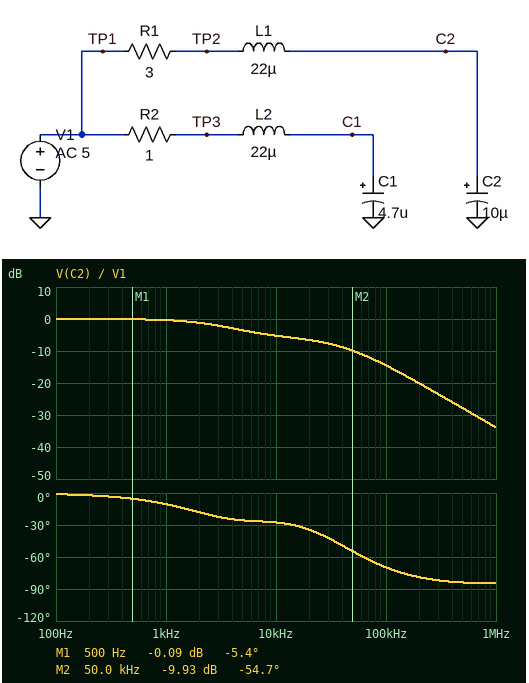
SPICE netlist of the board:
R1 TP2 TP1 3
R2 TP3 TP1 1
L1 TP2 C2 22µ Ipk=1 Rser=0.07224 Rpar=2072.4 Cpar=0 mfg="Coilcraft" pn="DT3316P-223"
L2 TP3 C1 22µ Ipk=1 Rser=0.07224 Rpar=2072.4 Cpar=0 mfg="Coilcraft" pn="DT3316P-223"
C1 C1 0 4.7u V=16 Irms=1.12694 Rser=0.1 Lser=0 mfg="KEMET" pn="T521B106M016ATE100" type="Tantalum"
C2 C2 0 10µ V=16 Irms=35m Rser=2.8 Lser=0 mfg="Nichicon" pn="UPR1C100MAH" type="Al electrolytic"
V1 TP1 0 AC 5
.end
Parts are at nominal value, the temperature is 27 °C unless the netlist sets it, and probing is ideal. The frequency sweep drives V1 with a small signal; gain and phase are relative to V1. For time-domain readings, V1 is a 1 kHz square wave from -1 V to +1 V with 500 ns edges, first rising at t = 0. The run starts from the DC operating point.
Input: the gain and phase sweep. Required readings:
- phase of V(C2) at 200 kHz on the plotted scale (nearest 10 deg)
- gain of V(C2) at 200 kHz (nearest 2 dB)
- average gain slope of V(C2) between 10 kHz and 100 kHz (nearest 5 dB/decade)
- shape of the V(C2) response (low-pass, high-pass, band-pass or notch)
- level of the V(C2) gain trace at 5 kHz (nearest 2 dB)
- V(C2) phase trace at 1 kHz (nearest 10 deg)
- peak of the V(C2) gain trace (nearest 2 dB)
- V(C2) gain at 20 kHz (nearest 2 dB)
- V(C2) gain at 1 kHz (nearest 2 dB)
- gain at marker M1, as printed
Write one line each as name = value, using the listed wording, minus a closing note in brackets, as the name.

phase of V(C2) at 200 kHz on the plotted scale = -80 deg
gain of V(C2) at 200 kHz = -20 dB
average gain slope of V(C2) between 10 kHz and 100 kHz = -10 dB/decade
shape of the V(C2) response = low-pass
level of the V(C2) gain trace at 5 kHz = -4 dB
V(C2) phase trace at 1 kHz = -10 deg
peak of the V(C2) gain trace = 0 dB
V(C2) gain at 20 kHz = -6 dB
V(C2) gain at 1 kHz = 0 dB
gain at marker M1, as printed = -0.09 dB
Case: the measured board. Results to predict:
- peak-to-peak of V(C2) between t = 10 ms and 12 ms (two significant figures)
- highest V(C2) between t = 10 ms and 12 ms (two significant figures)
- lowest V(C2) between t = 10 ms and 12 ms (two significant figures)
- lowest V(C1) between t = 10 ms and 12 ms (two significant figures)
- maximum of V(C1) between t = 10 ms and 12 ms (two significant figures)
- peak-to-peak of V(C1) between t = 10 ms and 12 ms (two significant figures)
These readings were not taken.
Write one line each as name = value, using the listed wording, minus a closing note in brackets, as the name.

peak-to-peak of V(C2) between t = 10 ms and 12 ms = 2.0 V
highest V(C2) between t = 10 ms and 12 ms = 1.0 V
lowest V(C2) between t = 10 ms and 12 ms = -1.0 V
lowest V(C1) between t = 10 ms and 12 ms = -1.8 V
maximum of V(C1) between t = 10 ms and 12 ms = 1.8 V
peak-to-peak of V(C1) between t = 10 ms and 12 ms = 3.7 V
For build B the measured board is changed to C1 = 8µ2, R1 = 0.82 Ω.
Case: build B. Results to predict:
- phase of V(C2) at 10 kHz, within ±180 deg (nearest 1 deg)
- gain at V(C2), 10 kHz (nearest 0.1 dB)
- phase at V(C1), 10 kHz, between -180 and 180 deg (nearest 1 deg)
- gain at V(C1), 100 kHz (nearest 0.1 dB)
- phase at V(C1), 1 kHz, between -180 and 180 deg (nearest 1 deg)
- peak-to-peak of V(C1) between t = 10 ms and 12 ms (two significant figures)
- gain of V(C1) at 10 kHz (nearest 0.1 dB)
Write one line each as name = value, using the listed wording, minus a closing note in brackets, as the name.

phase of V(C2) at 10 kHz, within ±180 deg = -26 deg
gain at V(C2), 10 kHz = -1.2 dB
phase at V(C1), 10 kHz, between -180 and 180 deg = -62 deg
gain at V(C1), 100 kHz = -35.9 dB
phase at V(C1), 1 kHz, between -180 and 180 deg = -3 deg
peak-to-peak of V(C1) between t = 10 ms and 12 ms = 3.2 V
gain of V(C1) at 10 kHz = 3.5 dB
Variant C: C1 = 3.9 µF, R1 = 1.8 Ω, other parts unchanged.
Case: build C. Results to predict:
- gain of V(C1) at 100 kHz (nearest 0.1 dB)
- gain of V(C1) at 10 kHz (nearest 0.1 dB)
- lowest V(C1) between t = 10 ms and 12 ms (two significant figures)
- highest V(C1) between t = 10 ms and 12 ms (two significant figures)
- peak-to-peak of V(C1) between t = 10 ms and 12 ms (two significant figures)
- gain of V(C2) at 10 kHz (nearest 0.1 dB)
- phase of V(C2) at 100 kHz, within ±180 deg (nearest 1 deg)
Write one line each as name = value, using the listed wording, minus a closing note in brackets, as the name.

gain of V(C1) at 100 kHz = -30.1 dB
gain of V(C1) at 10 kHz = 2.8 dB
lowest V(C1) between t = 10 ms and 12 ms = -1.9 V
highest V(C1) between t = 10 ms and 12 ms = 1.9 V
peak-to-peak of V(C1) between t = 10 ms and 12 ms = 3.8 V
gain of V(C2) at 10 kHz = -3.2 dB
phase of V(C2) at 100 kHz, within ±180 deg = -74 deg
